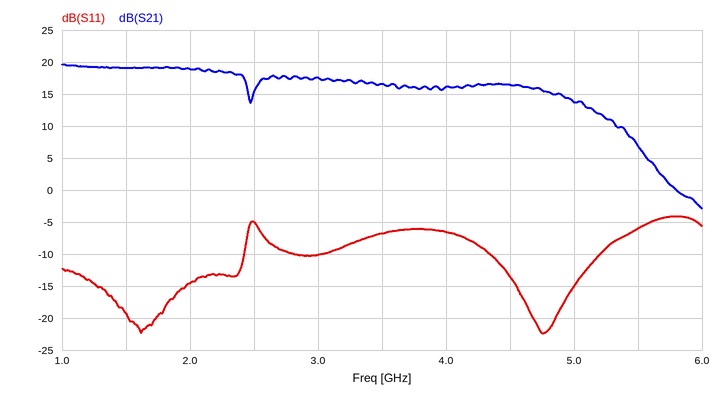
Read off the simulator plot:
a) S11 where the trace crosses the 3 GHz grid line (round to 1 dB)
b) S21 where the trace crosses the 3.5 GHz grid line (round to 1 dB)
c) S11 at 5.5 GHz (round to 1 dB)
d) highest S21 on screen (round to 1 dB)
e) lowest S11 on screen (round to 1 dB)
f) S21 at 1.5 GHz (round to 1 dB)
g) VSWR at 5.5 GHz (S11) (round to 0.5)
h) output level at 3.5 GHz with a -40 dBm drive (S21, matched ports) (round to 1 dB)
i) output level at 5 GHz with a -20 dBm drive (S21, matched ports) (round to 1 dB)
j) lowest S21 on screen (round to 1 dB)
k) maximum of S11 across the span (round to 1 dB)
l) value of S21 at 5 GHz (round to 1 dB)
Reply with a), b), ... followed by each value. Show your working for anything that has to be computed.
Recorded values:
a) -10 dB
b) 17 dB
c) -6 dB
d) 20 dB
e) -22 dB
f) 19 dB
g) |Γ| = 10^(-6/20) = 0.5012; VSWR = (1 + 0.5012)/(1 − 0.5012) ≈ 3.0
h) -40 dBm + (17 dB) = -23 dBm
i) -20 dBm + (14 dB) = -6 dBm
j) -3 dB
k) -4 dB
l) 14 dB
